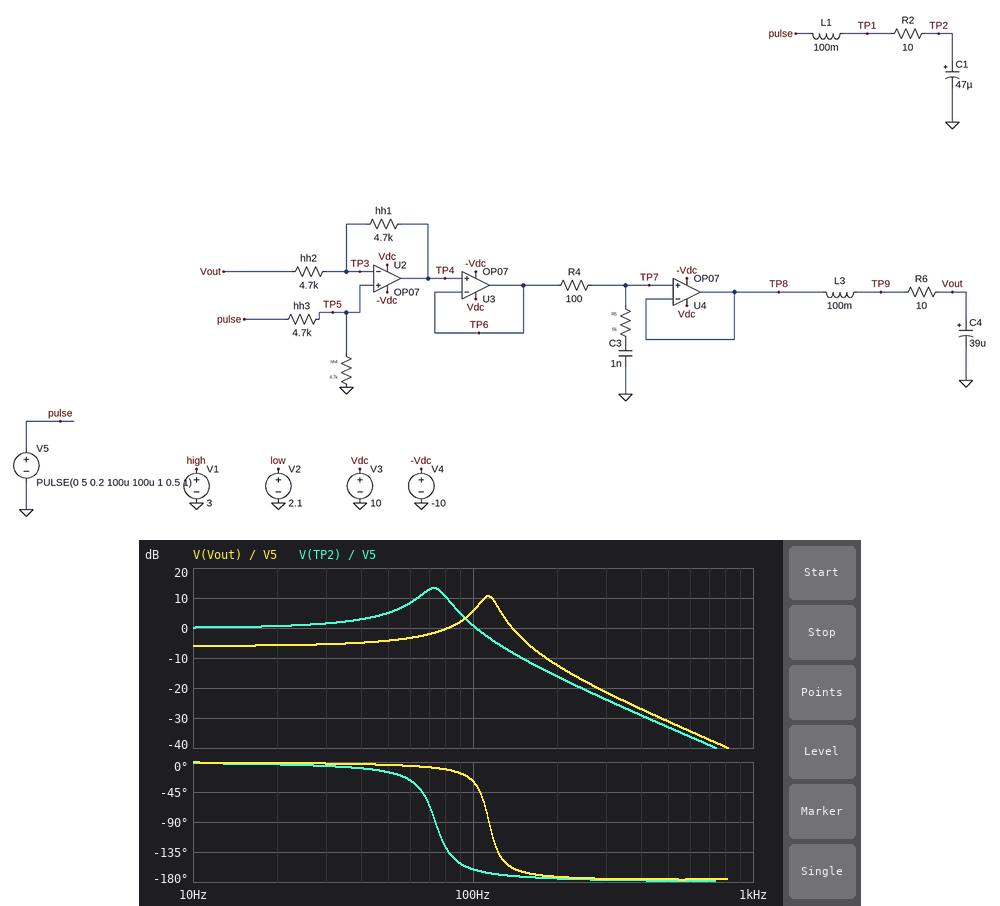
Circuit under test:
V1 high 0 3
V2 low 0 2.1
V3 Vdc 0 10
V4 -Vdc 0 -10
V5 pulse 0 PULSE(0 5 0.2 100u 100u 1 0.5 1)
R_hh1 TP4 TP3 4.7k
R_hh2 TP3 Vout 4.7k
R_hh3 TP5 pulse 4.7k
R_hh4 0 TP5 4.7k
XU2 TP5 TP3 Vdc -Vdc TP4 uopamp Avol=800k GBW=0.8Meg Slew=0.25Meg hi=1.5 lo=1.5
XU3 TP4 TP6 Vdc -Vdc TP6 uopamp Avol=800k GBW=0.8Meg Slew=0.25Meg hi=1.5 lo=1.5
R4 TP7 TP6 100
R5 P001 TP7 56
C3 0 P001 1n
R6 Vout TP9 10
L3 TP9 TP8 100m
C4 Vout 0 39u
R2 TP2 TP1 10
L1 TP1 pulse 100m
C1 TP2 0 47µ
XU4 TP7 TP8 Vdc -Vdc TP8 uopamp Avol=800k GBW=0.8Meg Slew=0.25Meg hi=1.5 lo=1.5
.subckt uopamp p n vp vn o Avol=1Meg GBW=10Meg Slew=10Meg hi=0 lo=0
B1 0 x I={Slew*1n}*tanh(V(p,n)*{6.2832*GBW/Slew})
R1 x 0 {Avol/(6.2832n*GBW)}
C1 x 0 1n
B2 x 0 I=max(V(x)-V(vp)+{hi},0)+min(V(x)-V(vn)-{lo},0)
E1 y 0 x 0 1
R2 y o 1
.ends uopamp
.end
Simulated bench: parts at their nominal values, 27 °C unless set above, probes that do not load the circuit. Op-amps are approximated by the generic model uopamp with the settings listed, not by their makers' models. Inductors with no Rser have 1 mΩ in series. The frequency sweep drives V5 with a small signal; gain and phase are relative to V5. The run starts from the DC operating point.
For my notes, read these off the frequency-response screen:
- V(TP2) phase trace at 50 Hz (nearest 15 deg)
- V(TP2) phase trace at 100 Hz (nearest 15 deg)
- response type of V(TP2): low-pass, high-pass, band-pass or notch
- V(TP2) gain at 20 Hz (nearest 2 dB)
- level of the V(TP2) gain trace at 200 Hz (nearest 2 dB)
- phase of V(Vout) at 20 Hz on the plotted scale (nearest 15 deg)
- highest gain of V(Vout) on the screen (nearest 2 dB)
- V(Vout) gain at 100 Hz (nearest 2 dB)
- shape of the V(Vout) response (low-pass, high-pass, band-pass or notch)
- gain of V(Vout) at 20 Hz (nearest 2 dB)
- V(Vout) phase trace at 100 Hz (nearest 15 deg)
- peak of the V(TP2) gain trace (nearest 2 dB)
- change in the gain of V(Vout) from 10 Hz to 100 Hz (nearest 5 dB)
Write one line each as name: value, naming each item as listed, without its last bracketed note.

V(TP2) phase trace at 50 Hz: -15 deg
V(TP2) phase trace at 100 Hz: -165 deg
response type of V(TP2): low-pass, high-pass, band-pass or notch: low-pass
V(TP2) gain at 20 Hz: 0 dB
level of the V(TP2) gain trace at 200 Hz: -16 dB
phase of V(Vout) at 20 Hz on the plotted scale: 0 deg
highest gain of V(Vout) on the screen: 10 dB
V(Vout) gain at 100 Hz: 6 dB
shape of the V(Vout) response: low-pass
gain of V(Vout) at 20 Hz: -6 dB
V(Vout) phase trace at 100 Hz: -30 deg
peak of the V(TP2) gain trace: 14 dB
change in the gain of V(Vout) from 10 Hz to 100 Hz: 10 dB
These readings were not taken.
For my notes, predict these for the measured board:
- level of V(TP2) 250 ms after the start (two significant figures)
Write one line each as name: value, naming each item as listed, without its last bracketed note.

level of V(TP2) 250 ms after the start: 5.3 V
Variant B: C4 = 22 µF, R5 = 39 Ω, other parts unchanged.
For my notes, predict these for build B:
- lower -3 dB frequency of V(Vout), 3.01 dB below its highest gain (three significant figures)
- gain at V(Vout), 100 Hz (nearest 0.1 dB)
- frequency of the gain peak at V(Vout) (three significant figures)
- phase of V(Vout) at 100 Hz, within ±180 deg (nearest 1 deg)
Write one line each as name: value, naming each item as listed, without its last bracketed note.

lower -3 dB frequency of V(Vout), 3.01 dB below its highest gain: 142 Hz
gain at V(Vout), 100 Hz: -1.2 dB
frequency of the gain peak at V(Vout): 151 Hz
phase of V(Vout) at 100 Hz, within ±180 deg: -7 deg
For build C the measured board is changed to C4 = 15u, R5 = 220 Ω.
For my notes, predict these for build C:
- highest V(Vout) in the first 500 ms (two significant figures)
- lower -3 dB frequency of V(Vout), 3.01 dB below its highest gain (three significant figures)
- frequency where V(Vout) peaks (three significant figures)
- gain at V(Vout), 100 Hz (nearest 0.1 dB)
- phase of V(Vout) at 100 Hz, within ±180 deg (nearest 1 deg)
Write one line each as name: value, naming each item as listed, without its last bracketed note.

highest V(Vout) in the first 500 ms: 4.6 V
lower -3 dB frequency of V(Vout), 3.01 dB below its highest gain: 174 Hz
frequency where V(Vout) peaks: 183 Hz
gain at V(Vout), 100 Hz: -3.0 dB
phase of V(Vout) at 100 Hz, within ±180 deg: -4 deg
